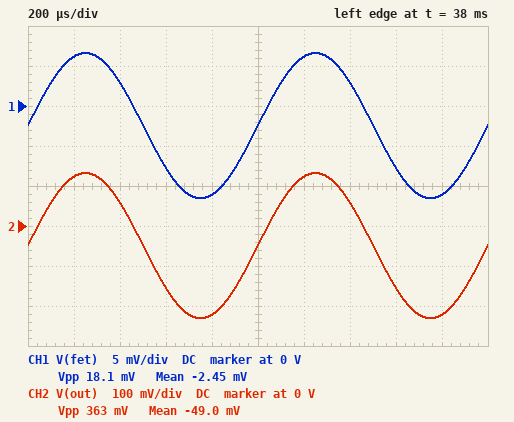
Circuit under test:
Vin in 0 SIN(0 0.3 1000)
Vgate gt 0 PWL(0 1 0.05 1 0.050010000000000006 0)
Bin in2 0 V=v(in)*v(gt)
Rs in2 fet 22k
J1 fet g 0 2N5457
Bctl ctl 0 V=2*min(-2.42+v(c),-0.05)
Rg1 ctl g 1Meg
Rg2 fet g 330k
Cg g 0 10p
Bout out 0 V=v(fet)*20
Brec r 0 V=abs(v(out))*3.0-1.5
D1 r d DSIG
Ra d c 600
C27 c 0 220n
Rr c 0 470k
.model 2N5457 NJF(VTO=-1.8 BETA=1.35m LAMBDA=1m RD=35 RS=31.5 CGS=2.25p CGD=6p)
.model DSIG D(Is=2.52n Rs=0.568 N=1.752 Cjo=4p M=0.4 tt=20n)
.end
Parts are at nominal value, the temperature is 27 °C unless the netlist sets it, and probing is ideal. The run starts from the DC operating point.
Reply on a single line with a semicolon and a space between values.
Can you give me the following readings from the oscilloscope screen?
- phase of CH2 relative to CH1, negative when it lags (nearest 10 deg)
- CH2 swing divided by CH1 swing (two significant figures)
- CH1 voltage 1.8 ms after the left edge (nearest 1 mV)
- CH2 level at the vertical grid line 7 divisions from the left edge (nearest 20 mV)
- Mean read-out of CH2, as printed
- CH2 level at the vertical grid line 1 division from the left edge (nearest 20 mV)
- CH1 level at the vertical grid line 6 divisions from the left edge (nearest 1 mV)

0 deg; 20; -11 mV; 60 mV; -49.0 mV; 120 mV; 6 mV
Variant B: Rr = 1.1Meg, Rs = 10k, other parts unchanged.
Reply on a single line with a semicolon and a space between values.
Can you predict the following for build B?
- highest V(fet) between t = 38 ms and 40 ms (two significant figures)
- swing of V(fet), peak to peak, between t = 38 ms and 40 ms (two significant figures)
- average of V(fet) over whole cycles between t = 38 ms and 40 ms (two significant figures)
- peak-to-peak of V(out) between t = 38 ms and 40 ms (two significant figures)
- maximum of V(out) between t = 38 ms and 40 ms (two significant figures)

17 mV; 39 mV; -2.4 mV; 770 mV; 340 mV
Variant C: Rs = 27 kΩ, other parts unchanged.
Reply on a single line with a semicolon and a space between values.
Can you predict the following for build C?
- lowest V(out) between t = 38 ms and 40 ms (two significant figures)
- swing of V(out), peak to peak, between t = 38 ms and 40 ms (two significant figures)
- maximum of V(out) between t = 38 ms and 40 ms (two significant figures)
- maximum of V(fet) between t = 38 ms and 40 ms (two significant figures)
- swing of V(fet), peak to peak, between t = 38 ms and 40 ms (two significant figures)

-200 mV; 300 mV; 100 mV; 5.0 mV; 15 mV
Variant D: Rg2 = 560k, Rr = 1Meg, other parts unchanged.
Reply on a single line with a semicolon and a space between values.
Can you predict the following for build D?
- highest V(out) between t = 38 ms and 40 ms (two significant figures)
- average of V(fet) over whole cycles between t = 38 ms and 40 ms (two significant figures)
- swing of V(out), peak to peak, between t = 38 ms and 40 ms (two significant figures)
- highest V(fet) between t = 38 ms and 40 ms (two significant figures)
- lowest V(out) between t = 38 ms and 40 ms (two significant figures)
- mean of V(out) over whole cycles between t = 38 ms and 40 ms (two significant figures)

410 mV; -5.9 mV; 1.1 V; 21 mV; -660 mV; -120 mV
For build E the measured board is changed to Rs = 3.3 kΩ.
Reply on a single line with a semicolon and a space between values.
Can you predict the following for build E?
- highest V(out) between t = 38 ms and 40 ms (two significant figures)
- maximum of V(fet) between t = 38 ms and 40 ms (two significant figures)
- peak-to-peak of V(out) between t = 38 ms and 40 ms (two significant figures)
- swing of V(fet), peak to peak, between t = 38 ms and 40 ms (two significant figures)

750 mV; 38 mV; 1.6 V; 78 mV
